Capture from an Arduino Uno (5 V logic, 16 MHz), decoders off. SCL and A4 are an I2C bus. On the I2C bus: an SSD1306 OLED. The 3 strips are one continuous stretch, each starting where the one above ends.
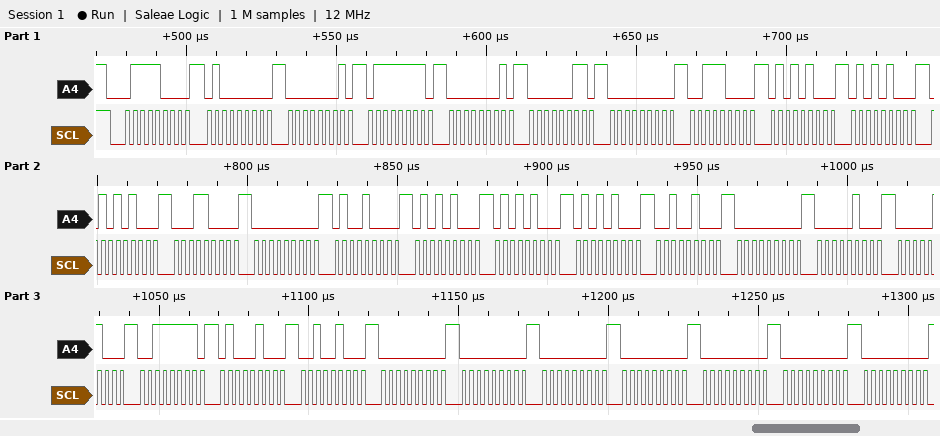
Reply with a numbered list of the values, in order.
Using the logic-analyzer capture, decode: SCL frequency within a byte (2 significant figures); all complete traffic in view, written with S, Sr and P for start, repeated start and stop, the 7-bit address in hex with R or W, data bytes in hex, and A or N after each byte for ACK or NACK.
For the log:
1. 400 kHz
2. S 3CW A 40 A 01 A 7F A 01 A 03 A 00 A 38 A 54 A 54 A 54 A 18 A 00 A 48 A 54 A 54 A 54 A 24 A 00 A 04 A 04 A 3F A 44 A 24 A 00 A 00 A 00 A 00 A 00 A 00 A 00 A
